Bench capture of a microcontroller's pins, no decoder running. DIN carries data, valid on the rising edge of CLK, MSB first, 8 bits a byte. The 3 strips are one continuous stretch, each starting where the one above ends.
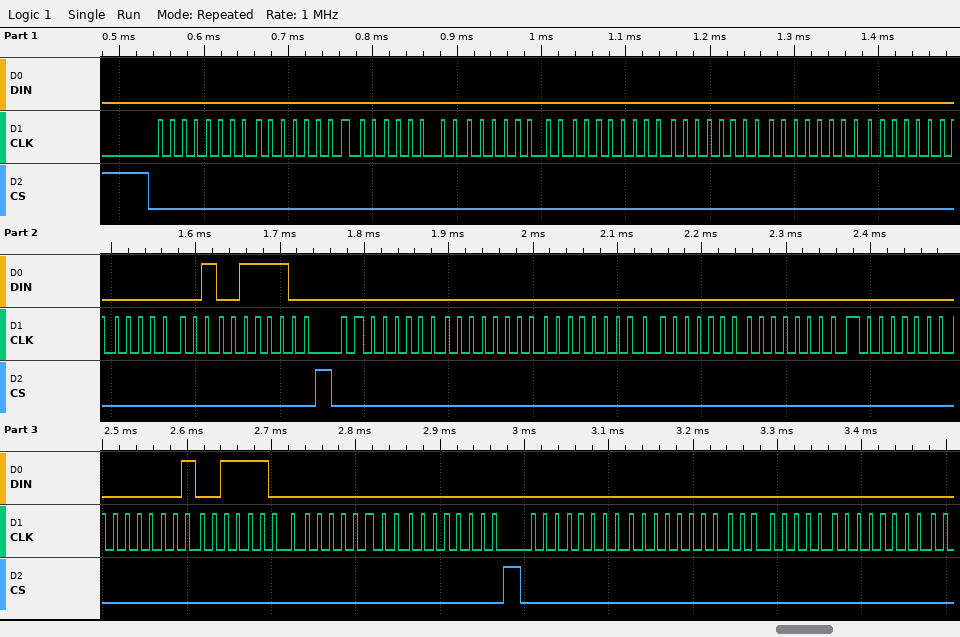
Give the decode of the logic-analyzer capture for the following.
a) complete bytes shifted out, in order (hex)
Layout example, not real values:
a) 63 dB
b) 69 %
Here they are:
a) 00 00 00 00 00 00 00 00 01 3C 00 00 00 00 00 00 01 3C 00 00 00 00 00 00
